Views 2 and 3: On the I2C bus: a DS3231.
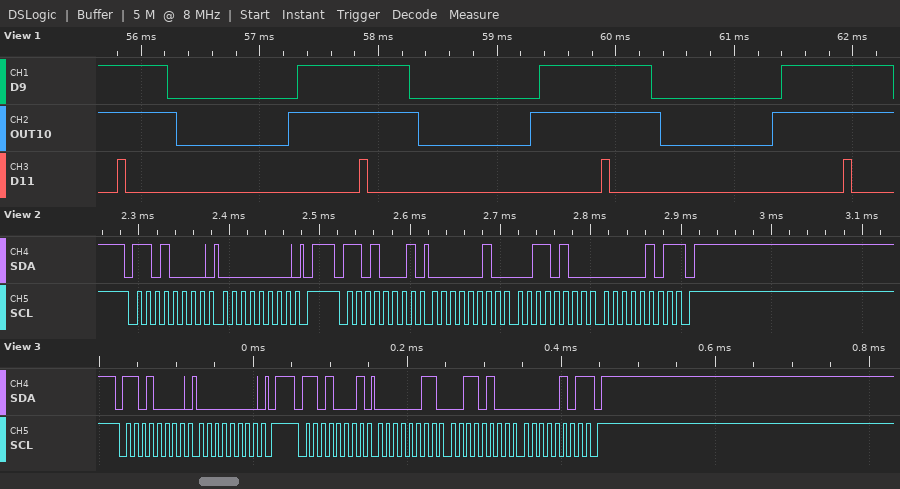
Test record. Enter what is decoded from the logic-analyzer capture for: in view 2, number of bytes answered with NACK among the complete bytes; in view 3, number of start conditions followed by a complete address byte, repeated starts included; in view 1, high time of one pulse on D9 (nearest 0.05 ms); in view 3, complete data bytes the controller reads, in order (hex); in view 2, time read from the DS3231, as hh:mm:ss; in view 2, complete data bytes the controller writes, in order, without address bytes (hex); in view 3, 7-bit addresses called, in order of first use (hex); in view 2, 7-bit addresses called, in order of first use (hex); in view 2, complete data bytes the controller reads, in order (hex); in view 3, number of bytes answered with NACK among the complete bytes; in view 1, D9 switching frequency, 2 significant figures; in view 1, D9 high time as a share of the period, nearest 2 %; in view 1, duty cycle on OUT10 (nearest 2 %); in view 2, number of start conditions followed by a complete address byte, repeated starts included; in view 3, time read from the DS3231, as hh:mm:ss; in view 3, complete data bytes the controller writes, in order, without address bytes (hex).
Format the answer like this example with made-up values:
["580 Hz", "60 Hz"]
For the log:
["1", "2", "0.95 ms", "03 34 05", "05:34:02", "00", "0x68", "0x68", "02 34 05", "1", "490 Hz", "46 %", "54 %", "2", "05:34:03", "00"]
